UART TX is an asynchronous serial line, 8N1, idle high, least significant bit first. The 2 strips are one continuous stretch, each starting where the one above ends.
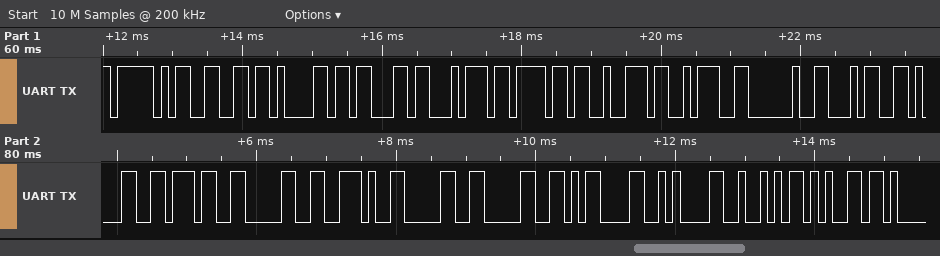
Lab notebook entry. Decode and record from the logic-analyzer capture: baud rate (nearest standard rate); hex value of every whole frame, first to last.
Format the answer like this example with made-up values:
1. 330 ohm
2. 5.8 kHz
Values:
1. 9600 baud
2. 0x5F 0x66 0x61 0x63 0x74 0x6F 0x72 0x3A 0x20 0x34 0x31 0x37 0x30 0x2E 0x30 0x30 0x0D 0x0A 0x52 0x65
